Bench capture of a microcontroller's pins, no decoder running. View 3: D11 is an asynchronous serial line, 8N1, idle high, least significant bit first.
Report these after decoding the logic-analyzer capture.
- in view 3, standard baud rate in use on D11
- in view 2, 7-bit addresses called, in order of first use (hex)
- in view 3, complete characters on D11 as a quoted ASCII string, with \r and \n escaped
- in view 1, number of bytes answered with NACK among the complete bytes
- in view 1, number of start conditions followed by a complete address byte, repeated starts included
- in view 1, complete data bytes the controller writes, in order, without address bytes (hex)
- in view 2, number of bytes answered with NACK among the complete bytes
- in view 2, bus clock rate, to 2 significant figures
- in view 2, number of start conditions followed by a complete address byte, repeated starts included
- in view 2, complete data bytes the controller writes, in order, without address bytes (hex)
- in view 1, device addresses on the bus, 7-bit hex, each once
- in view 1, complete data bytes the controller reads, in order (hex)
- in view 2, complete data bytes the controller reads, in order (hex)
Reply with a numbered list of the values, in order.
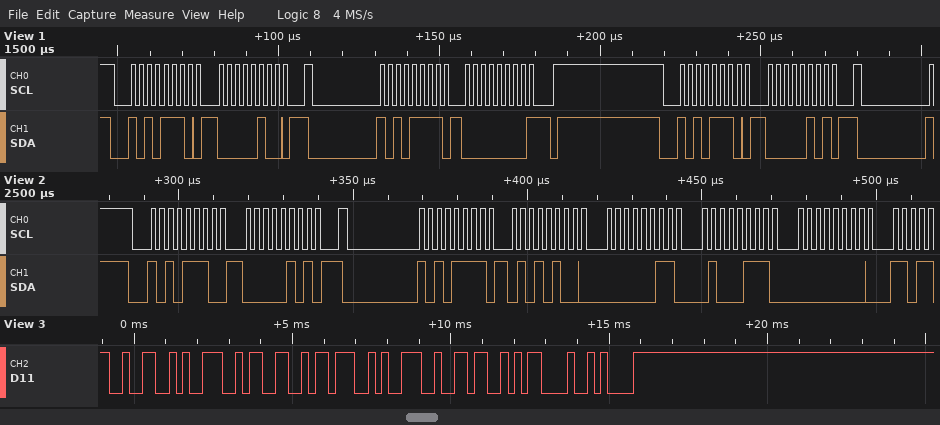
1. 4800 baud
2. 0x57
3. "293;96\r\n"
4. 1
5. 3
6. 04 05
7. 0
8. 400 kHz
9. 2
10. 05
11. 0x57
12. 00
13. 54 03 47 00
